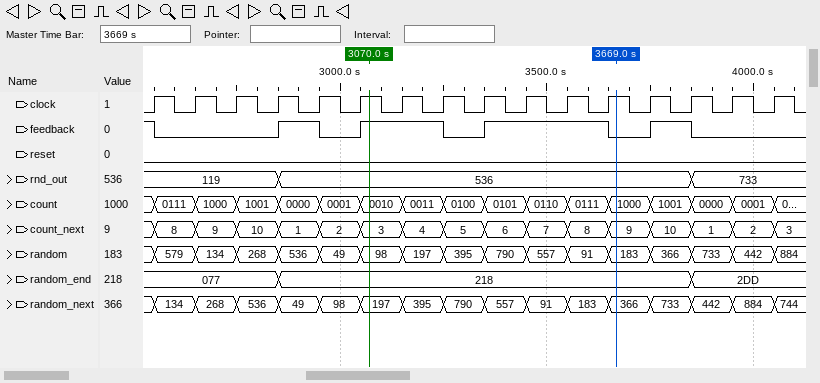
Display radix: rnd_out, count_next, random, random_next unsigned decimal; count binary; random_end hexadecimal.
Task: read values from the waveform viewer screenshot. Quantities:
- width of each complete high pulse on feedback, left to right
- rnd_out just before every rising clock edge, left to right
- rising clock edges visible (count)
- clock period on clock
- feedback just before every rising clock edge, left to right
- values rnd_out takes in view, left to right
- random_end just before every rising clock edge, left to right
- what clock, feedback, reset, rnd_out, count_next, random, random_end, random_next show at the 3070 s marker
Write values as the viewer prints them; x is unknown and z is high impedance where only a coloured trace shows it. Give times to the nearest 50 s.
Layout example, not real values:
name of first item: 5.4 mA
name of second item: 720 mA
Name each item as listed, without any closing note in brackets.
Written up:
width of each complete high pulse on feedback, left to right: 100 s, 200 s, 300 s, 100 s
rnd_out just before every rising clock edge, left to right: 119, 119, 119, 119, 536, 536, 536, 536, 536, 536, 536, 536, 536, 536, 733, 733
rising clock edges visible: 16
clock period on clock: 100 s
feedback just before every rising clock edge, left to right: 1 0 0 0 1 0 1 1 0 1 1 1 0 1 0 0
values rnd_out takes in view, left to right: 119, 536, 733
random_end just before every rising clock edge, left to right: 077, 077, 077, 077, 218, 218, 218, 218, 218, 218, 218, 218, 218, 218, 2DD, 2DD
what clock, feedback, reset, rnd_out, count_next, random, random_end, random_next show at the 3070 s marker: clock=1, feedback=1, reset=0, rnd_out=536, count_next=3, random=98, random_end=218, random_next=197
